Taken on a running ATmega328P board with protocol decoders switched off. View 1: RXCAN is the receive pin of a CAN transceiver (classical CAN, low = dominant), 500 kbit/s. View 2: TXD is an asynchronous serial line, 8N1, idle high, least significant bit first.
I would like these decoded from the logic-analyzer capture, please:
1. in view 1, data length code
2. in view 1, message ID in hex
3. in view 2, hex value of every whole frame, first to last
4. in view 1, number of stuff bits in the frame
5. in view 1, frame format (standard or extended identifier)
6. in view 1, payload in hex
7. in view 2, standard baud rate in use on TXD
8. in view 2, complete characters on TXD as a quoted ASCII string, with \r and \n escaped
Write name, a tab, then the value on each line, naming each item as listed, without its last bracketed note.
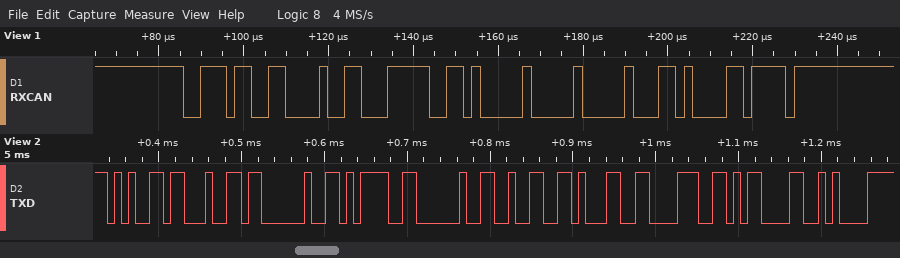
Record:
in view 1, data length code	4
in view 1, message ID in hex	0x3B3
in view 2, hex value of every whole frame, first to last	65 64 20 3D 20 32 31 38 0D 0A
in view 1, number of stuff bits in the frame	4
in view 1, frame format	standard
in view 1, payload in hex	C7 DA 00 00
in view 2, standard baud rate in use on TXD	115200 baud
in view 2, complete characters on TXD as a quoted ASCII string, with \r and \n escaped	"ed = 218\r\n"
